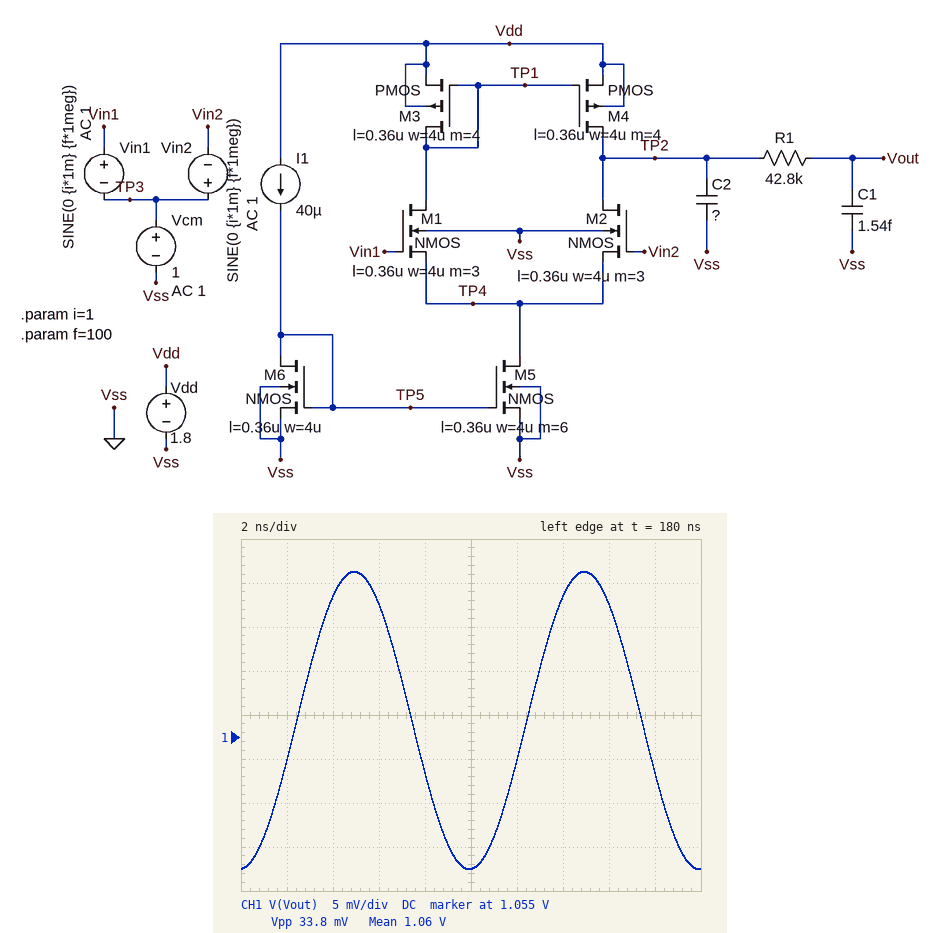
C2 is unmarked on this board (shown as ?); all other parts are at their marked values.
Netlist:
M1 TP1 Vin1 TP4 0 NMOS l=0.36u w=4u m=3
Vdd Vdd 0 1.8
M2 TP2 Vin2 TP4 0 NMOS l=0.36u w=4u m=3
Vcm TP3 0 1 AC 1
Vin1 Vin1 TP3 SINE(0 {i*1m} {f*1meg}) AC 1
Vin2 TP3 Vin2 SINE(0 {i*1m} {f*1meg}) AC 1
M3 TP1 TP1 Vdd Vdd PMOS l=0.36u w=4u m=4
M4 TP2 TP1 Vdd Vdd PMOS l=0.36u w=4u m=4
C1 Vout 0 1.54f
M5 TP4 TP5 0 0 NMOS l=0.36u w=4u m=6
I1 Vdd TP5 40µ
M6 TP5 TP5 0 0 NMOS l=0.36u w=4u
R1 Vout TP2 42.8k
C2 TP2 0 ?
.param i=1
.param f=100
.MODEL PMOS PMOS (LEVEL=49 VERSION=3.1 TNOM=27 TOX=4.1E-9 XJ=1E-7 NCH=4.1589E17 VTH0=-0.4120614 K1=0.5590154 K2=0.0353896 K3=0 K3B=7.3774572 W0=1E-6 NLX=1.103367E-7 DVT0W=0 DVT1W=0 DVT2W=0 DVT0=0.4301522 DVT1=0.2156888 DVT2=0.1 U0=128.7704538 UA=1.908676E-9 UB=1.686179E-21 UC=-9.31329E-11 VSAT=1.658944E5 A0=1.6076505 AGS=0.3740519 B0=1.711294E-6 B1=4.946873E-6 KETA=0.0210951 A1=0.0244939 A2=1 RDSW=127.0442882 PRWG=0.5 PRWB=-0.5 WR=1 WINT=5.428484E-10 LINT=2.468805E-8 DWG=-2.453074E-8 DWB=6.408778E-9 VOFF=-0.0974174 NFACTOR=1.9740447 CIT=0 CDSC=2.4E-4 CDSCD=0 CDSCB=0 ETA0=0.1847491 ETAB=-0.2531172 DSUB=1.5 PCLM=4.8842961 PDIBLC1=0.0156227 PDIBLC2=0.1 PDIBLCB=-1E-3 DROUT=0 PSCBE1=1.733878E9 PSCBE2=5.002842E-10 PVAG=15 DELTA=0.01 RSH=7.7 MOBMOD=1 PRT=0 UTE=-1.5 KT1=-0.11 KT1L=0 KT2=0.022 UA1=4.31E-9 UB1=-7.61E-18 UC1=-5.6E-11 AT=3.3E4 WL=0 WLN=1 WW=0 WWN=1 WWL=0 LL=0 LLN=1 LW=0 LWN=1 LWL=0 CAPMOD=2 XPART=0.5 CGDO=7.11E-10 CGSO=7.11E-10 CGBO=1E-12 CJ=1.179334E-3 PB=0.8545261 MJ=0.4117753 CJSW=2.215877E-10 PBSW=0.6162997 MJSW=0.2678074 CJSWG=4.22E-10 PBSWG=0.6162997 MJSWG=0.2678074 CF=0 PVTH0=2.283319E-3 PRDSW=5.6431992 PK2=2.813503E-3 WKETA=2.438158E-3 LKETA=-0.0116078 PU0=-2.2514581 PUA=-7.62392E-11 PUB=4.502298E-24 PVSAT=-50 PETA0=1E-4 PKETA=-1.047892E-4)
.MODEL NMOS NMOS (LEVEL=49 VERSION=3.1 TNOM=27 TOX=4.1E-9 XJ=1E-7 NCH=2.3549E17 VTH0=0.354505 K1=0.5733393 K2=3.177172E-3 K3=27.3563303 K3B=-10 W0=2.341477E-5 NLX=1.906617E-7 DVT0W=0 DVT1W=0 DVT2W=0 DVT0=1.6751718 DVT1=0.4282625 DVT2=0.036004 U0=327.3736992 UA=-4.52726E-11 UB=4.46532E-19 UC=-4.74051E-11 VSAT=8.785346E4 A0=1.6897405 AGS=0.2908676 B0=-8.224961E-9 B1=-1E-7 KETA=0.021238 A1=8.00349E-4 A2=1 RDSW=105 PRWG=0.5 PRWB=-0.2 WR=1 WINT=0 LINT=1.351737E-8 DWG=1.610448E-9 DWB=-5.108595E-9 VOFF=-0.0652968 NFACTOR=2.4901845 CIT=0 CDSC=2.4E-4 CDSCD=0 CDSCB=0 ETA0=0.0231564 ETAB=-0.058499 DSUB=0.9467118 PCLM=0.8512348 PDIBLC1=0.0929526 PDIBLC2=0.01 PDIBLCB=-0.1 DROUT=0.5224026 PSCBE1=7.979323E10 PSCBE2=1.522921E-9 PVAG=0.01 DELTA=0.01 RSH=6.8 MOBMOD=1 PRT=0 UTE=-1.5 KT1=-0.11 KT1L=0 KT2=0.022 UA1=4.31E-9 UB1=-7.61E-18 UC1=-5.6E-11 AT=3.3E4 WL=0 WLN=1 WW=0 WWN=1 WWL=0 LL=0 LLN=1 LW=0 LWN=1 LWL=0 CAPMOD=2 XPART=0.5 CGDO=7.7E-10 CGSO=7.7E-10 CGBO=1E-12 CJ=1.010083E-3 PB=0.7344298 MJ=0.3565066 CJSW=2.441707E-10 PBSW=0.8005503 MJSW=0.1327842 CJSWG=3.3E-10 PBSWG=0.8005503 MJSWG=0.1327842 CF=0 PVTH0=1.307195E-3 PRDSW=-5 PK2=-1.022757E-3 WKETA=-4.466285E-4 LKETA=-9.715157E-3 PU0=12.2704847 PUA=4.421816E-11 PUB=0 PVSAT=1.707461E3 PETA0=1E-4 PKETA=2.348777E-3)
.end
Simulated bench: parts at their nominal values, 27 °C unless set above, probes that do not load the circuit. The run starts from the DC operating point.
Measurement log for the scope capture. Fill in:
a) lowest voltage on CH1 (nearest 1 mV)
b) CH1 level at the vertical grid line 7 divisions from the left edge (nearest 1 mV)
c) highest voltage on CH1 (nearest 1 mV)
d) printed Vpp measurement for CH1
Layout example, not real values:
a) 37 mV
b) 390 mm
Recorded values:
a) 1.040 V
b) 1.071 V
c) 1.074 V
d) 33.8 mV
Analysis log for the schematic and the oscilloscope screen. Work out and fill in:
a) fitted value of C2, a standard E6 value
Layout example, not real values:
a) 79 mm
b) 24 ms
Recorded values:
a) 220 fF
